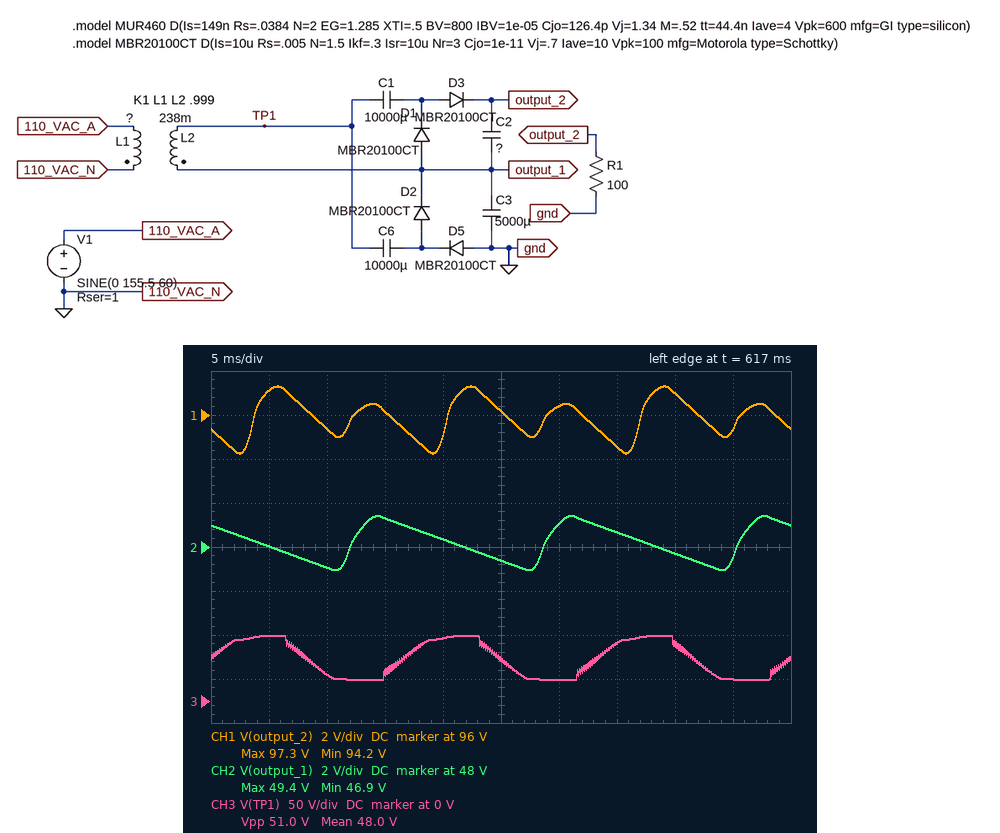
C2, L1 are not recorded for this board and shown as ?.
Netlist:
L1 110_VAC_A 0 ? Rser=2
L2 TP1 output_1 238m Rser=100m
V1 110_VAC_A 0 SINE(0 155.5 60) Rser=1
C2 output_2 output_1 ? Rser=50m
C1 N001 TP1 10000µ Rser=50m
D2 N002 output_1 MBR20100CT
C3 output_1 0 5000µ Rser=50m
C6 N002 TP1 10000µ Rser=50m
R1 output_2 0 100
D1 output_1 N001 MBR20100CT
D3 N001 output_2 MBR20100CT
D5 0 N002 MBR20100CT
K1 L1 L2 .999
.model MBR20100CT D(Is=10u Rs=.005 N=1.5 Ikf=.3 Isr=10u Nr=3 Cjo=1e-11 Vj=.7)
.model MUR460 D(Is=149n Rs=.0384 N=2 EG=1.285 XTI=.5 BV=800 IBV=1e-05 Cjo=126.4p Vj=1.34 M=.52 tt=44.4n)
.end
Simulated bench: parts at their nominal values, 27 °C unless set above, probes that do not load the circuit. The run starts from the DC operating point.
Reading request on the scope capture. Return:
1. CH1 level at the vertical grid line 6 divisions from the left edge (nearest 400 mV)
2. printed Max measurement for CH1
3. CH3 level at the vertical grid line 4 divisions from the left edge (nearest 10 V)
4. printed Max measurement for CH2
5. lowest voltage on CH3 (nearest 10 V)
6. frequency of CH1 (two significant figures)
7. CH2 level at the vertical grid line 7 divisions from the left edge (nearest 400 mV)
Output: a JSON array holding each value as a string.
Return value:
["96.4 V", "97.3 V", "70 V", "49.4 V", "20 V", "120 Hz", "48.8 V"]
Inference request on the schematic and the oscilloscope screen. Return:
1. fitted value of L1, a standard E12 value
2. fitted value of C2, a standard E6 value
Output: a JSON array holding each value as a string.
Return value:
["6.8 H", "3.3 mF"]
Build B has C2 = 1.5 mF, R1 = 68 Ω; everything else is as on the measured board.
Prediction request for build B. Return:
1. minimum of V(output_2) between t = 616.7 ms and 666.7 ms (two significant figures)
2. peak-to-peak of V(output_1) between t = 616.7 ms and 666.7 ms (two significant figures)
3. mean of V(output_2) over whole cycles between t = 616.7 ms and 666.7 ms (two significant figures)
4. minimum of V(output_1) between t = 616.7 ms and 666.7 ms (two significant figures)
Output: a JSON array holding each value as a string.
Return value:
["87 V", "3.4 V", "92 V", "46 V"]
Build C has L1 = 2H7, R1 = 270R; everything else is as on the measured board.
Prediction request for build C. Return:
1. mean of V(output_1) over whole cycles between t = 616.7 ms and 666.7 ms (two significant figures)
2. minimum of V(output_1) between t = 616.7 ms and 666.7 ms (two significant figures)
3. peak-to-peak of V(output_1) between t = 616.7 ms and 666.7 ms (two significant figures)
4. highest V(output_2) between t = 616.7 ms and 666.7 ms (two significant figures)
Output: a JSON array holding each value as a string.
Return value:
["81 V", "80 V", "1.6 V", "160 V"]
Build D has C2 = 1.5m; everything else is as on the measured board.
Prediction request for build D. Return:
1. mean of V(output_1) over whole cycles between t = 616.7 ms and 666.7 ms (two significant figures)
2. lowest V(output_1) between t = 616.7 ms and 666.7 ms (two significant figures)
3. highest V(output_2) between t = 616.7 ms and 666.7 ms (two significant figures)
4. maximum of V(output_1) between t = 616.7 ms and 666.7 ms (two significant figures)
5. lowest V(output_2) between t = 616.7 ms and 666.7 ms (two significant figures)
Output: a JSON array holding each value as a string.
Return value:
["49 V", "48 V", "100 V", "51 V", "92 V"]
